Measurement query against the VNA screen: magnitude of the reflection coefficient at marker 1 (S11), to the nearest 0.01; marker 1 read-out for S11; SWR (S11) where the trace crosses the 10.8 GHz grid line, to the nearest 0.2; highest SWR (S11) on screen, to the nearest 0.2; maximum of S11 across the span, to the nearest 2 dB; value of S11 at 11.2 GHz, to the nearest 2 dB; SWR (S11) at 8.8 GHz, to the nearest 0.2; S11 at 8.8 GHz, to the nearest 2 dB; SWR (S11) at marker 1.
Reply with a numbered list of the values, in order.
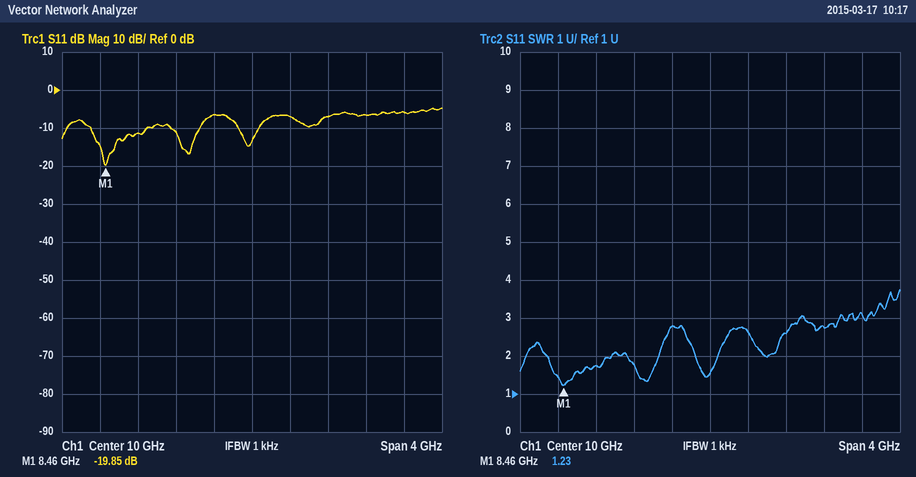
1. 0.10
2. -19.85 dB
3. 2.6
4. 3.8
5. -4 dB
6. -6 dB
7. 1.8
8. -12 dB
9. 1.23
